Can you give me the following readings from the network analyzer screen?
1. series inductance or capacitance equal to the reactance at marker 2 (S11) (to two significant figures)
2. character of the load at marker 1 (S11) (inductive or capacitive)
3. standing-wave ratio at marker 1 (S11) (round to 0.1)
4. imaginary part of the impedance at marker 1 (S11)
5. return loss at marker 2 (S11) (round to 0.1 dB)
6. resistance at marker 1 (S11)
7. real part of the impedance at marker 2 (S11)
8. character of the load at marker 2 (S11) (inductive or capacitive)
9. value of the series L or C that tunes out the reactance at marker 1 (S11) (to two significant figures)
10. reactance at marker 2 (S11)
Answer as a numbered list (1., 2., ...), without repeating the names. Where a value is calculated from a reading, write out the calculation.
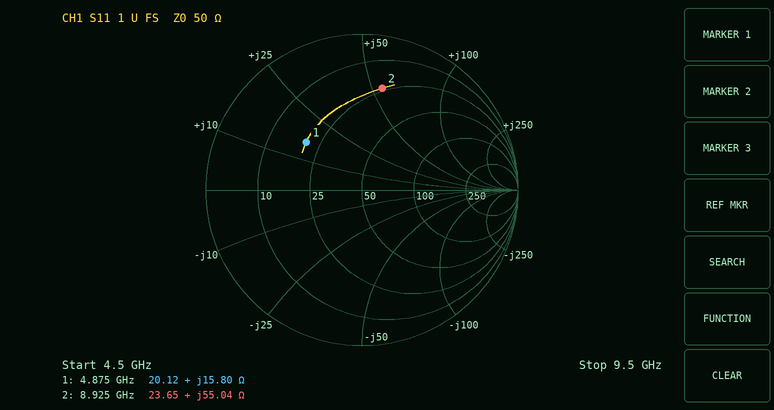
1. L = 55.04 Ω/(2π × 8.925 GHz) ≈ 982 pH, so 980 pH to two significant figures
2. inductive
3. 2.8
4. +15.80 Ω
5. 3.6 dB
6. 20.12 Ω
7. 23.65 Ω
8. inductive
9. C = 1/(2π × 4.875 GHz × 15.8 Ω) ≈ 2.1 pF
10. +55.04 Ω
